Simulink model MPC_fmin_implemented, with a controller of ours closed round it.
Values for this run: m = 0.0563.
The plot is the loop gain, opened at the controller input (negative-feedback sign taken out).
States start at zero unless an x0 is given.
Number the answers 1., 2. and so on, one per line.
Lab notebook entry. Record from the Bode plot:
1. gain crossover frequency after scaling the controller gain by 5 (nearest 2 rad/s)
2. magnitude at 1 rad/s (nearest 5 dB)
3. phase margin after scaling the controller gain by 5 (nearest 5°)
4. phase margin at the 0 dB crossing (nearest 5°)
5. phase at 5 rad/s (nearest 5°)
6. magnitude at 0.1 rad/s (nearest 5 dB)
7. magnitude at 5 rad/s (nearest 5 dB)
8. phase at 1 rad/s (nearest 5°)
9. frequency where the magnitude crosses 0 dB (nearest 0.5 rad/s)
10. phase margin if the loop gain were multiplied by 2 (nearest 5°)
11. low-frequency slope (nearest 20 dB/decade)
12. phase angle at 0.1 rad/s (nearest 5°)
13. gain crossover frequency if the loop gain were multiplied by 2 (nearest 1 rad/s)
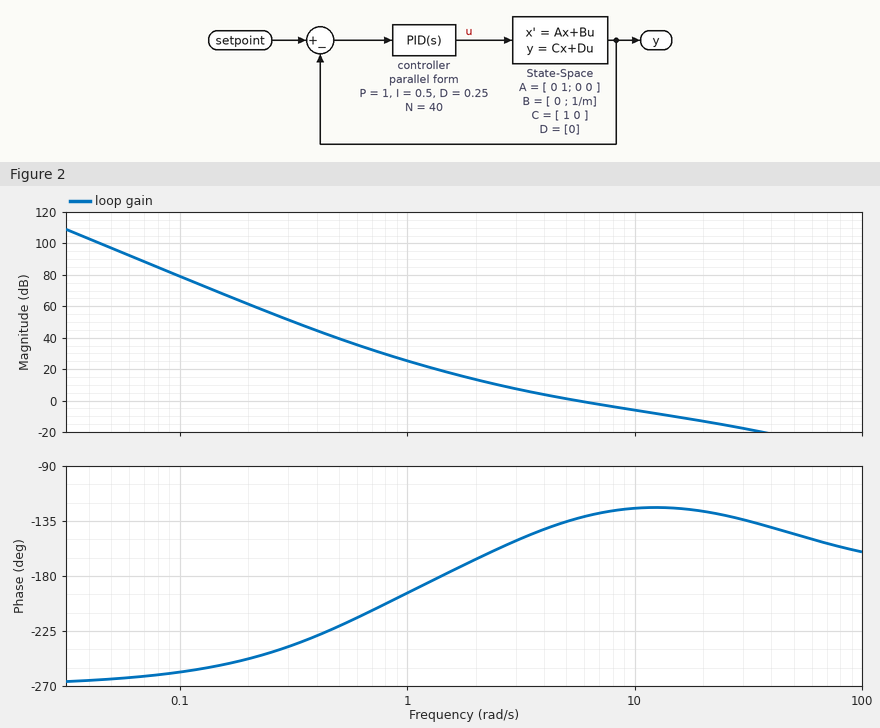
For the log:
1. 22 rad/s
2. 25 dB
3. 50°
4. 45°
5. -135°
6. 80 dB
7. 0 dB
8. -195°
9. 5.5 rad/s
10. 55°
11. -60 dB/decade
12. -260°
13. 10 rad/s
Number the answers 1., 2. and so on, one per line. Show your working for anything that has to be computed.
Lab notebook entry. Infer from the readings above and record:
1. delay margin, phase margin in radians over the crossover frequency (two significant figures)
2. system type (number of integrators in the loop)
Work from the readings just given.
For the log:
1. 45 × π / 180 / 5.5 = 0.14 s
2. 3
